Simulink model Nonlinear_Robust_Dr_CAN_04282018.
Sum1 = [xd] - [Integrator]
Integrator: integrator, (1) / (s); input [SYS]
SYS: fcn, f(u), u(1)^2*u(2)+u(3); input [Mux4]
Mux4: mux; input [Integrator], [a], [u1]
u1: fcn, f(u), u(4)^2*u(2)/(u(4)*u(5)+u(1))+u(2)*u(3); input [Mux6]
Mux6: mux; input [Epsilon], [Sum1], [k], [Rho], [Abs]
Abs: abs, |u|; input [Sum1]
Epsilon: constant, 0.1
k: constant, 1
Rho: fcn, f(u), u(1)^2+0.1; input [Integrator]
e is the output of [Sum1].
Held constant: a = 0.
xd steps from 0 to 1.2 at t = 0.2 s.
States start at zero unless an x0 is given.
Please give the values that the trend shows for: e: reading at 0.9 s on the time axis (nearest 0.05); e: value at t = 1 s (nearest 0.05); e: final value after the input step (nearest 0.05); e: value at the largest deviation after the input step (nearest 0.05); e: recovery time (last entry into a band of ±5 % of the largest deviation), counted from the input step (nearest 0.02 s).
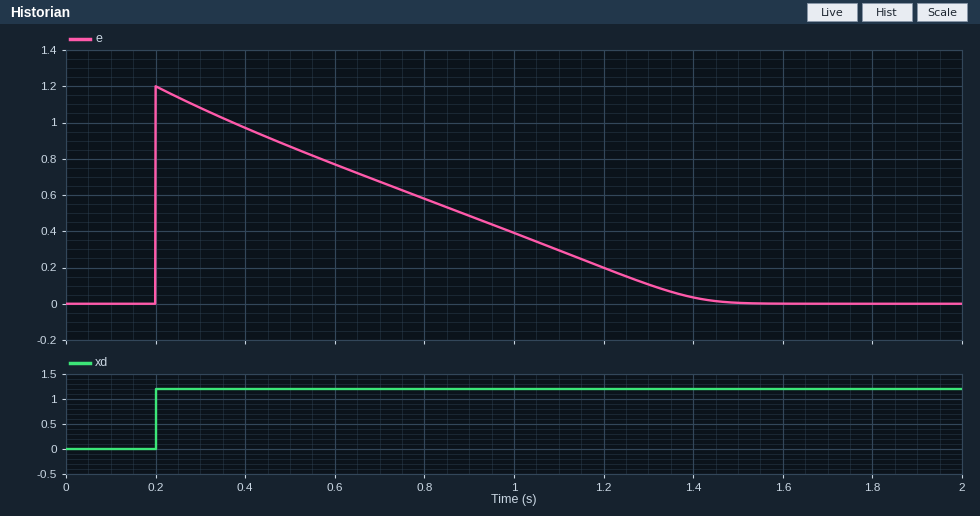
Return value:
0.50
0.40
0.00
1.20
1.16 s
